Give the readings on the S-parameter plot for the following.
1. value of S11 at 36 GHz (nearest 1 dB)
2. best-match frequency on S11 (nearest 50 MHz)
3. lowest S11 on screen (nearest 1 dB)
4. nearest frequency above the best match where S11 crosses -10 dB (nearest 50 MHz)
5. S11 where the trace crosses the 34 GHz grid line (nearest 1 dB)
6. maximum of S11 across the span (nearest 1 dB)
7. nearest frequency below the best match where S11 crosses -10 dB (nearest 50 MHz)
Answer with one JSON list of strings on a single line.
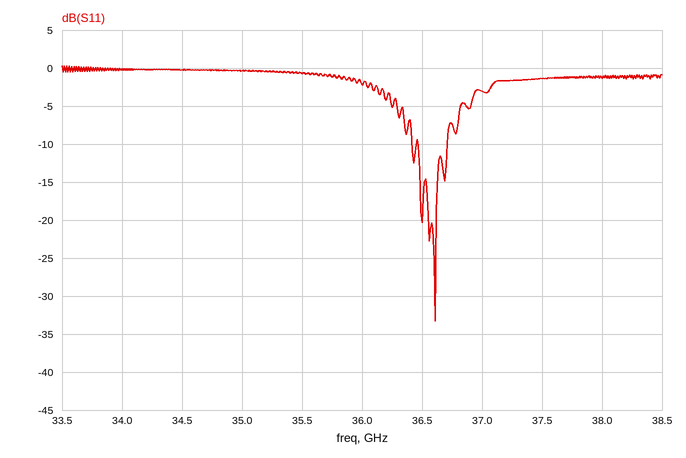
["-2 dB", "36.60 GHz", "-33 dB", "36.70 GHz", "0 dB", "0 dB", "36.45 GHz"]
